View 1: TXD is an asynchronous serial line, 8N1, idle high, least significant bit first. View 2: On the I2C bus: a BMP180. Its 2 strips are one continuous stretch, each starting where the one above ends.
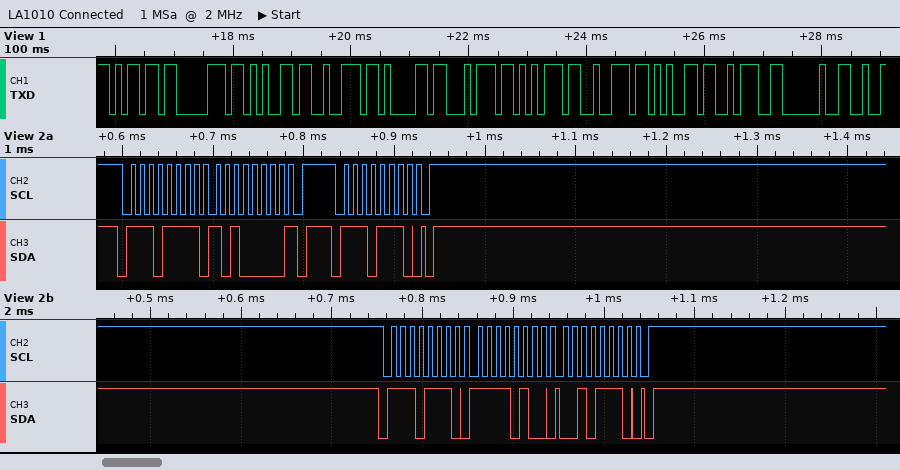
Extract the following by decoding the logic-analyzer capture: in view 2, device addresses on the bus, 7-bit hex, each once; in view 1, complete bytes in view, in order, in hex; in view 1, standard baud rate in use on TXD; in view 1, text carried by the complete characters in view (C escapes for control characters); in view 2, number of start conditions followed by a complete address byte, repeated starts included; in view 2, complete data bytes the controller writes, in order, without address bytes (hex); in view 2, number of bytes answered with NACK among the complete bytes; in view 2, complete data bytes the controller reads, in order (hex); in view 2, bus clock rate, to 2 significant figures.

0x77
0x6D 0x70 0x65 0x72 0x61 0x74 0x75 0x72 0x65 0x3A 0x20
9600 baud
"mperature: "
3
F4 2E
1
A0
100 kHz
